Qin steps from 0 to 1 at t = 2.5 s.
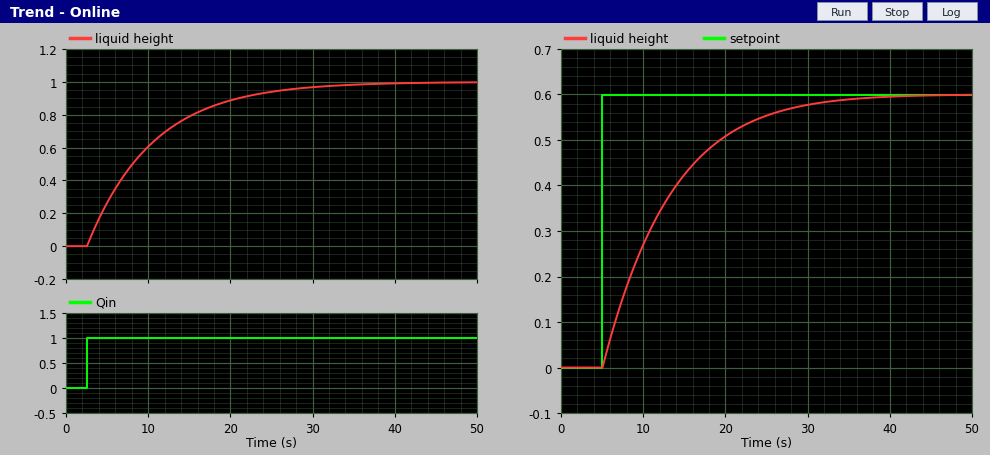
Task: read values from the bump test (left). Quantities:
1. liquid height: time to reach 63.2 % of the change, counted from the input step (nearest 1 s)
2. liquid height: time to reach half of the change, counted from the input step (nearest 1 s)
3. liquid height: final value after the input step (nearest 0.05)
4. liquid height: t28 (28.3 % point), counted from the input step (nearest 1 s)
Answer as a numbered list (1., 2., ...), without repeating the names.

1. 8 s
2. 6 s
3. 1.00
4. 3 s
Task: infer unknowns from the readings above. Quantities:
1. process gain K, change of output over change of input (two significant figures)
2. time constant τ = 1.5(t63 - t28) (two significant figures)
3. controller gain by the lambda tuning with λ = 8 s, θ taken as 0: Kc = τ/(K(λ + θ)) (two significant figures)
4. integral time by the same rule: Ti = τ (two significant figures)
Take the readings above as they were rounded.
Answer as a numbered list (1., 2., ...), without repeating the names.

1. 1.0
2. 7.5 s
3. 0.94
4. 7.5 s
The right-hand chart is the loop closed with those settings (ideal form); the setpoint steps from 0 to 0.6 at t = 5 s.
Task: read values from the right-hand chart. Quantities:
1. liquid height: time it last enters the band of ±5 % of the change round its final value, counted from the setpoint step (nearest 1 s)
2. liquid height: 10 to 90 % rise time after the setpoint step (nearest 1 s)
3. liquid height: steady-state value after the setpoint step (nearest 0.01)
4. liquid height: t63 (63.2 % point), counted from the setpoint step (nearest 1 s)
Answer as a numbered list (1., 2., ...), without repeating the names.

1. 23 s
2. 17 s
3. 0.60
4. 8 s
